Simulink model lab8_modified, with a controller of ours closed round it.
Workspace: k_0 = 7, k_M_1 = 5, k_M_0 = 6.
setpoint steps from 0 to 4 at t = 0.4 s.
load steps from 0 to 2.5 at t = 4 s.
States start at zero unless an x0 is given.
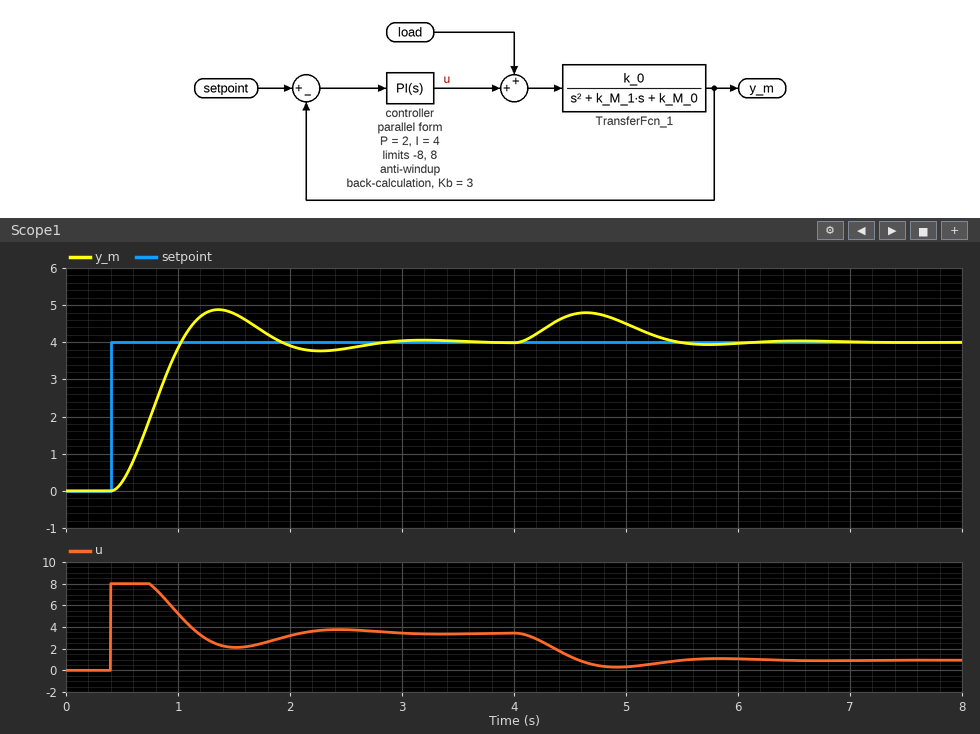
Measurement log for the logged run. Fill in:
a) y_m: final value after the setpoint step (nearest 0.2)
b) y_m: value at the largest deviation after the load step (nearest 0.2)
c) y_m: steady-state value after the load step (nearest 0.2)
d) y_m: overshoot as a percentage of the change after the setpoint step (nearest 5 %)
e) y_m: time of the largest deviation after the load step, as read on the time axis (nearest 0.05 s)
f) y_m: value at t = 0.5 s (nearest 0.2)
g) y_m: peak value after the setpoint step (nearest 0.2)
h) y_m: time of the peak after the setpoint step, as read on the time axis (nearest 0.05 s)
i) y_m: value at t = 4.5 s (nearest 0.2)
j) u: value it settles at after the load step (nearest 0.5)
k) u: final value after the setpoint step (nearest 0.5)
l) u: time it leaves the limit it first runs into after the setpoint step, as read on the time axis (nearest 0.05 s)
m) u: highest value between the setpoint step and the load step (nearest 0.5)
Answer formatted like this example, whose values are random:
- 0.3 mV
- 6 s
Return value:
- 4.0
- 4.8
- 4.0
- 20 %
- 4.65 s
- 0.2
- 4.8
- 1.35 s
- 4.8
- 1.0
- 3.5
- 0.75 s
- 8.0
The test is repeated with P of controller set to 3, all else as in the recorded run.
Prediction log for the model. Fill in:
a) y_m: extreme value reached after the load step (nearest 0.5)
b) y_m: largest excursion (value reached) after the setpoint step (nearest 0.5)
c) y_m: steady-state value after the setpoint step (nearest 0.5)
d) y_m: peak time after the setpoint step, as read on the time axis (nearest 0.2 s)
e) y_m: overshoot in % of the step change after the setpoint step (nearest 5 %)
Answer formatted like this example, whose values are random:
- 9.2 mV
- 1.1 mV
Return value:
- 4.5
- 4.5
- 4.0
- 1.2 s
- 10 %
